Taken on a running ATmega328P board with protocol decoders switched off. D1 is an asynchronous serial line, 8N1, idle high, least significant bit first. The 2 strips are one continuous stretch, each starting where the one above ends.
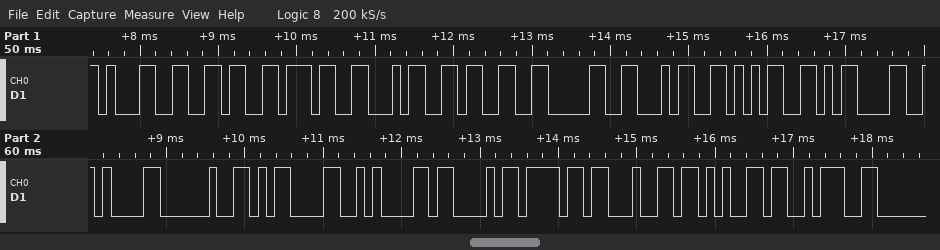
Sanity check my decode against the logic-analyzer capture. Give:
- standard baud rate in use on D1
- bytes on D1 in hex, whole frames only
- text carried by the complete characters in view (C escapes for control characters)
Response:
9600 baud
31 36 37 34 33 30 34 35 0D 0A 20 0D 0A 43 6F 64 65 3A
"16743045\r\n \r\nCode:"
